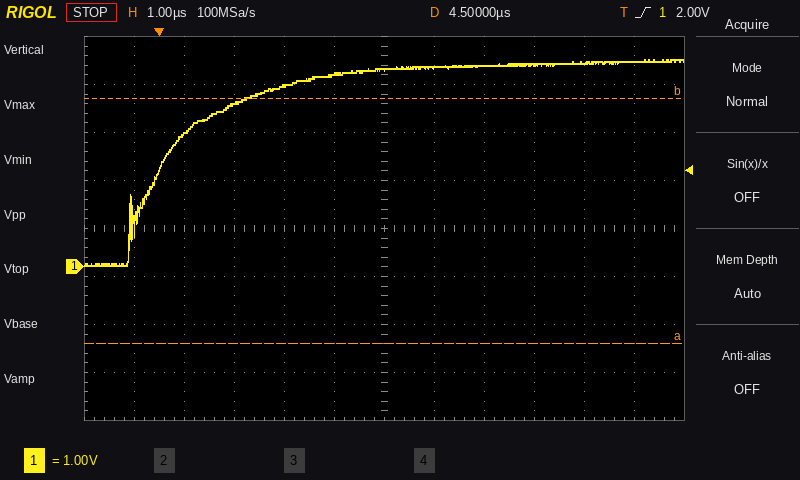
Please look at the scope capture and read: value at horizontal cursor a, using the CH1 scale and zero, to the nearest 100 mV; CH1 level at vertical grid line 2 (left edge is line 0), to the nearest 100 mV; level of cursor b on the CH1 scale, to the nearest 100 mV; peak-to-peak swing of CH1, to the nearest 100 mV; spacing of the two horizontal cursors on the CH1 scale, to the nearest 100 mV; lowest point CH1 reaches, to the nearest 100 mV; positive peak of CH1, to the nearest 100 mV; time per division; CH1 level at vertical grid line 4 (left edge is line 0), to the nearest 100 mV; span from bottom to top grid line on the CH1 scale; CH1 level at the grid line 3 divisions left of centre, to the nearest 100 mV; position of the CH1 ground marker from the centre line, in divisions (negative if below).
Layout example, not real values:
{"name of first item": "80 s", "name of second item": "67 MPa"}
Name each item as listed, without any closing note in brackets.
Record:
{"value at horizontal cursor a, using the CH1 scale and zero, to the nearest 100 mV": "-1.6 V", "CH1 level at vertical grid line 2 (left edge is line 0), to the nearest 100 mV": "2.8 V", "level of cursor b on the CH1 scale, to the nearest 100 mV": "3.5 V", "peak-to-peak swing of CH1, to the nearest 100 mV": "4.3 V", "spacing of the two horizontal cursors on the CH1 scale, to the nearest 100 mV": "5.1 V", "lowest point CH1 reaches, to the nearest 100 mV": "0.0 V", "positive peak of CH1, to the nearest 100 mV": "4.3 V", "time per division": "1 µs", "CH1 level at vertical grid line 4 (left edge is line 0), to the nearest 100 mV": "3.8 V", "span from bottom to top grid line on the CH1 scale": "8 V", "CH1 level at the grid line 3 divisions left of centre, to the nearest 100 mV": "3.4 V", "position of the CH1 ground marker from the centre line, in divisions": "-0.8 div"}
